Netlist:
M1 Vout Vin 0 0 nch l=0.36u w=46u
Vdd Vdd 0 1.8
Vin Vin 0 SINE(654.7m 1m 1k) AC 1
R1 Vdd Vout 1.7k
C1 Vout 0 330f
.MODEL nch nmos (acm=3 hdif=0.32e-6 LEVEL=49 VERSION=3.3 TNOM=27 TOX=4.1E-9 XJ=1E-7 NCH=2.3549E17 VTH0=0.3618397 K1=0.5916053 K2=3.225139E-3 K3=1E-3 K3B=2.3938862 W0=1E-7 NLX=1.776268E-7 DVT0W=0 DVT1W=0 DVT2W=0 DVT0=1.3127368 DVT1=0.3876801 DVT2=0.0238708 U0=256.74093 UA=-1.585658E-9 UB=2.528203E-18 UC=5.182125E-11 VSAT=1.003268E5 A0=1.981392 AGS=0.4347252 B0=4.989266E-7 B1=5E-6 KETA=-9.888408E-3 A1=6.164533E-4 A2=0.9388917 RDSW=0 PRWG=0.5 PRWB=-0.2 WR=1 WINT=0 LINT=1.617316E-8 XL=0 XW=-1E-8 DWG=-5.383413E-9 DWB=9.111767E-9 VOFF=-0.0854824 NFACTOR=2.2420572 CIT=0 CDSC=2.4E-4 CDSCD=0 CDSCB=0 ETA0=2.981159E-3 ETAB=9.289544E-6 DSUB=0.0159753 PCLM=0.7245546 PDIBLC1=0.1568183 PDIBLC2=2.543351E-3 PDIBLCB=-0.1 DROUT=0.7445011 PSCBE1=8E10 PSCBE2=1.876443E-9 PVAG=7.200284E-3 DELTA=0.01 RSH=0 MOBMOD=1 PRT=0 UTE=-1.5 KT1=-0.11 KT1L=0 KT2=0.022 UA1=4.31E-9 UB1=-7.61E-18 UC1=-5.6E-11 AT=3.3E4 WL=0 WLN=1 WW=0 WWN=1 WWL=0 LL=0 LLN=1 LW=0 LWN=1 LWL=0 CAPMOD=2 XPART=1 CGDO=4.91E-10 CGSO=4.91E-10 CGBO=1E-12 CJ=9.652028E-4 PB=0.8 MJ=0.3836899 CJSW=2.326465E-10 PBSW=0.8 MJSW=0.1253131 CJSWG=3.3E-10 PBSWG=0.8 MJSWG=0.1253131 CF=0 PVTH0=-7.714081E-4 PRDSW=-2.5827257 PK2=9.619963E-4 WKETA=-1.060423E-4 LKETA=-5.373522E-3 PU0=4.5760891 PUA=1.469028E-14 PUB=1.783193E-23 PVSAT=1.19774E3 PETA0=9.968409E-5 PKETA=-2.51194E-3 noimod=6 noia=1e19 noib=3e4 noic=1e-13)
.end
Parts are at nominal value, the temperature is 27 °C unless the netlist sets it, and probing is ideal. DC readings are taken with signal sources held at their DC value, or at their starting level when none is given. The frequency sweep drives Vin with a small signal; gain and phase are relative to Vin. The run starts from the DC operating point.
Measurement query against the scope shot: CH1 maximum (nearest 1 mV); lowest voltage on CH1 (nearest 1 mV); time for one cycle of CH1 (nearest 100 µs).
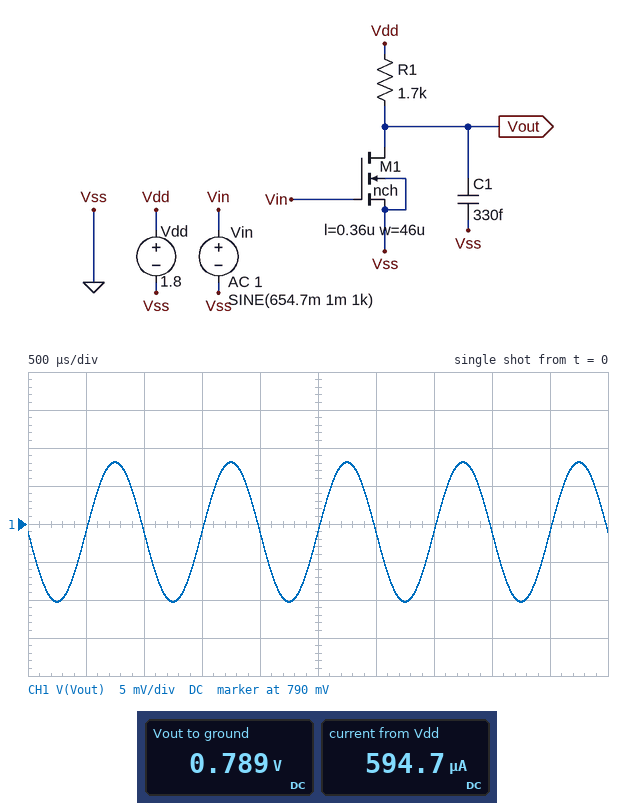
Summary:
798 mV
780 mV
1.0 ms
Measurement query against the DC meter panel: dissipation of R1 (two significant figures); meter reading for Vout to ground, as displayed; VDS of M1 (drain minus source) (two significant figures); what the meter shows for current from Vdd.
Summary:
600 µW
0.789 V
790 mV
594.7 µA
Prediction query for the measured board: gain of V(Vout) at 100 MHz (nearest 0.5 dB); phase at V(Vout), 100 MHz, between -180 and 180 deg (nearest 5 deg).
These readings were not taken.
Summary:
18.5 dB
160 deg
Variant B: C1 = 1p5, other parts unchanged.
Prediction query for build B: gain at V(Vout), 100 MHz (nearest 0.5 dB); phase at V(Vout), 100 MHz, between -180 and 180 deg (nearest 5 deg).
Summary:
14.0 dB
125 deg
